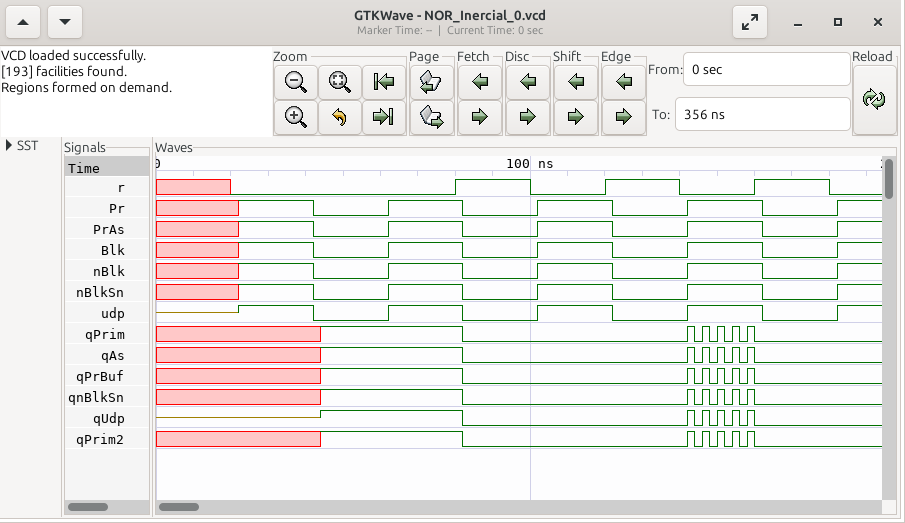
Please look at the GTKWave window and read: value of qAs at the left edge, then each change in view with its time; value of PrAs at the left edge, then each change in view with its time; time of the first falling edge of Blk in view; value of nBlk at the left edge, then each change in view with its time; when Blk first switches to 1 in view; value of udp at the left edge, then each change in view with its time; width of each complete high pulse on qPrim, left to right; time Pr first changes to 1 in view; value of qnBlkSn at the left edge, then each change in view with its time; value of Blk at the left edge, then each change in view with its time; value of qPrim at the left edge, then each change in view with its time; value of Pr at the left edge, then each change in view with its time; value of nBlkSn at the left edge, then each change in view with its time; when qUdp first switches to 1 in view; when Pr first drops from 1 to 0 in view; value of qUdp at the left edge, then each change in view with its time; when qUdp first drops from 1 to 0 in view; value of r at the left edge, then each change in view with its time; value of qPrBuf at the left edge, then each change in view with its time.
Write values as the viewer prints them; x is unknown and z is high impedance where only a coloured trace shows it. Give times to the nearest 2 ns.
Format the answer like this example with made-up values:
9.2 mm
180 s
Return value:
x, 1 at 44 ns, 0 at 82 ns, 1 at 142 ns, 0 at 144 ns, 1 at 146 ns, 0 at 148 ns, 1 at 150 ns, 0 at 152 ns, 1 at 154 ns, 0 at 156 ns, 1 at 158 ns, 0 at 160 ns
x, 1 at 22 ns, 0 at 42 ns, 1 at 62 ns, 0 at 82 ns, 1 at 102 ns, 0 at 122 ns, 1 at 142 ns, 0 at 162 ns, 1 at 182 ns
42 ns
x, 1 at 22 ns, 0 at 42 ns, 1 at 62 ns, 0 at 82 ns, 1 at 102 ns, 0 at 122 ns, 1 at 142 ns, 0 at 162 ns, 1 at 182 ns
22 ns
z, 1 at 22 ns, 0 at 42 ns, 1 at 62 ns, 0 at 82 ns, 1 at 102 ns, 0 at 122 ns, 1 at 142 ns, 0 at 162 ns, 1 at 182 ns
2 ns, 2 ns, 2 ns, 2 ns, 2 ns
22 ns
x, 1 at 44 ns, 0 at 82 ns, 1 at 142 ns, 0 at 144 ns, 1 at 146 ns, 0 at 148 ns, 1 at 150 ns, 0 at 152 ns, 1 at 154 ns, 0 at 156 ns, 1 at 158 ns, 0 at 160 ns
x, 1 at 22 ns, 0 at 42 ns, 1 at 62 ns, 0 at 82 ns, 1 at 102 ns, 0 at 122 ns, 1 at 142 ns, 0 at 162 ns, 1 at 182 ns
x, 1 at 44 ns, 0 at 82 ns, 1 at 142 ns, 0 at 144 ns, 1 at 146 ns, 0 at 148 ns, 1 at 150 ns, 0 at 152 ns, 1 at 154 ns, 0 at 156 ns, 1 at 158 ns, 0 at 160 ns
x, 1 at 22 ns, 0 at 42 ns, 1 at 62 ns, 0 at 82 ns, 1 at 102 ns, 0 at 122 ns, 1 at 142 ns, 0 at 162 ns, 1 at 182 ns
x, 1 at 22 ns, 0 at 42 ns, 1 at 62 ns, 0 at 82 ns, 1 at 102 ns, 0 at 122 ns, 1 at 142 ns, 0 at 162 ns, 1 at 182 ns
44 ns
42 ns
z, 1 at 44 ns, 0 at 82 ns, 1 at 142 ns, 0 at 144 ns, 1 at 146 ns, 0 at 148 ns, 1 at 150 ns, 0 at 152 ns, 1 at 154 ns, 0 at 156 ns, 1 at 158 ns, 0 at 160 ns
82 ns
x, 0 at 20 ns, 1 at 80 ns, 0 at 100 ns, 1 at 120 ns, 0 at 140 ns, 1 at 160 ns, 0 at 180 ns
x, 1 at 44 ns, 0 at 82 ns, 1 at 142 ns, 0 at 144 ns, 1 at 146 ns, 0 at 148 ns, 1 at 150 ns, 0 at 152 ns, 1 at 154 ns, 0 at 156 ns, 1 at 158 ns, 0 at 160 ns
